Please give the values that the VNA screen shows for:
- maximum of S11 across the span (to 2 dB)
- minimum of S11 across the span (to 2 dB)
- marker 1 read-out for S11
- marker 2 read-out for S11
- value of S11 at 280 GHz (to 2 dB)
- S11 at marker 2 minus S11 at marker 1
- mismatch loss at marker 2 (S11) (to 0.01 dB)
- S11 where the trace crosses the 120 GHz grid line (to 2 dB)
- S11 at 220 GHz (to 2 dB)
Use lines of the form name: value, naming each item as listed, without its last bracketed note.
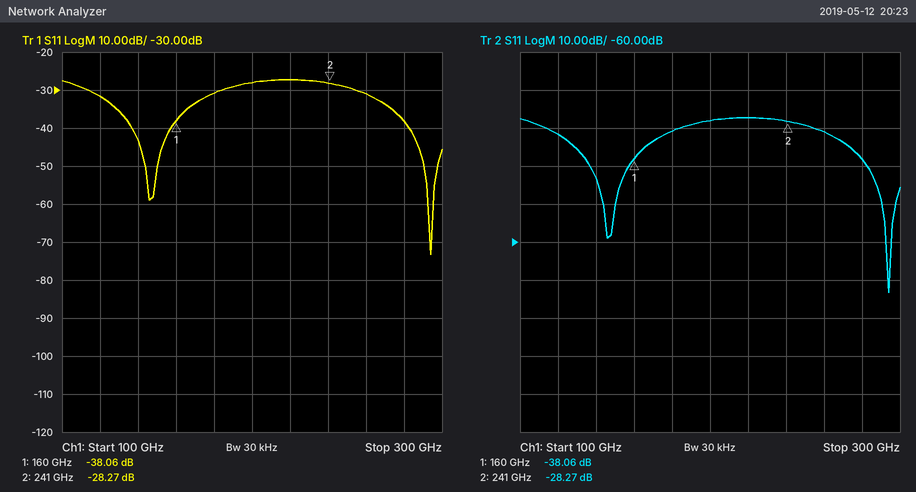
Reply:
maximum of S11 across the span: -28 dB
minimum of S11 across the span: -74 dB
marker 1 read-out for S11: -38.06 dB
marker 2 read-out for S11: -28.27 dB
value of S11 at 280 GHz: -38 dB
S11 at marker 2 minus S11 at marker 1: 9.79 dB
mismatch loss at marker 2 (S11): 0.01 dB
S11 where the trace crosses the 120 GHz grid line: -32 dB
S11 at 220 GHz: -28 dB
